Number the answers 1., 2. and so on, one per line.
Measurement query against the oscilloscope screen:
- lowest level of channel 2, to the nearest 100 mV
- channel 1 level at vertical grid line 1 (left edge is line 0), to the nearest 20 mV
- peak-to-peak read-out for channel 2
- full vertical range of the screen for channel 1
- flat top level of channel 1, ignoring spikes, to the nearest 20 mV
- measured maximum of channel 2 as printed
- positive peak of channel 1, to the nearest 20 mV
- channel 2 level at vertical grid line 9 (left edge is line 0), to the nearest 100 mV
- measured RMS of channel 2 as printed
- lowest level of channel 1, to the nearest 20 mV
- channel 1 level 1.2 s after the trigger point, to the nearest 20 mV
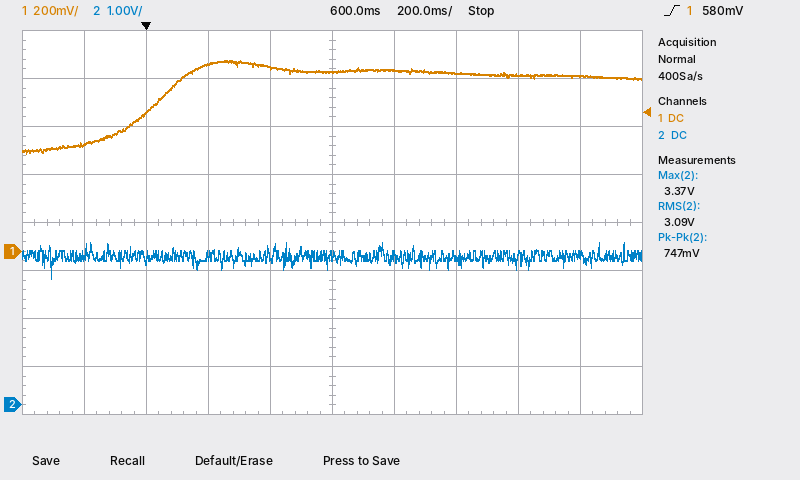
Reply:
1. 2.6 V
2. 440 mV
3. 747 mV
4. 1.6 V
5. 740 mV
6. 3.37 V
7. 800 mV
8. 3.1 V
9. 3.09 V
10. 400 mV
11. 740 mV
